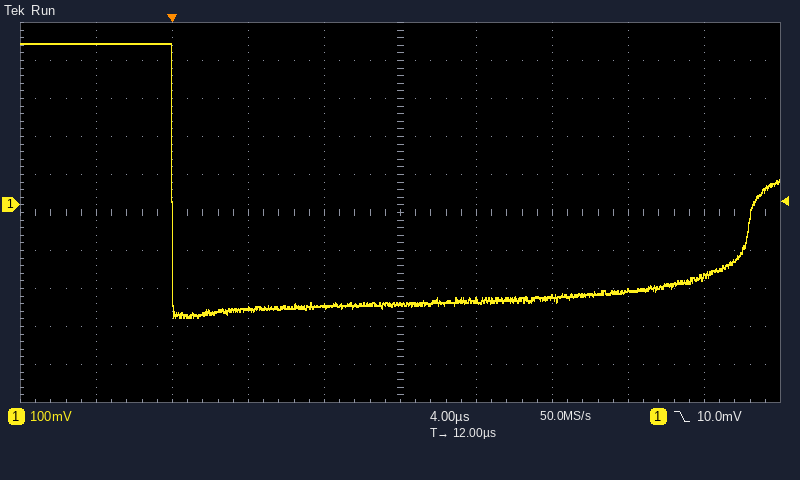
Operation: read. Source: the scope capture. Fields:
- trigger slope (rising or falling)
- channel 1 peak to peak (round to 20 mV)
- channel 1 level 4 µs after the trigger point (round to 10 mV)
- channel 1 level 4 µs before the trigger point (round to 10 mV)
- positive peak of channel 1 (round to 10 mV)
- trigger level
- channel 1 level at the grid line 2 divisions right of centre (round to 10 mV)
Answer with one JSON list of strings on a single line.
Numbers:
["falling", "720 mV", "-270 mV", "420 mV", "420 mV", "10.0 mV", "-240 mV"]
